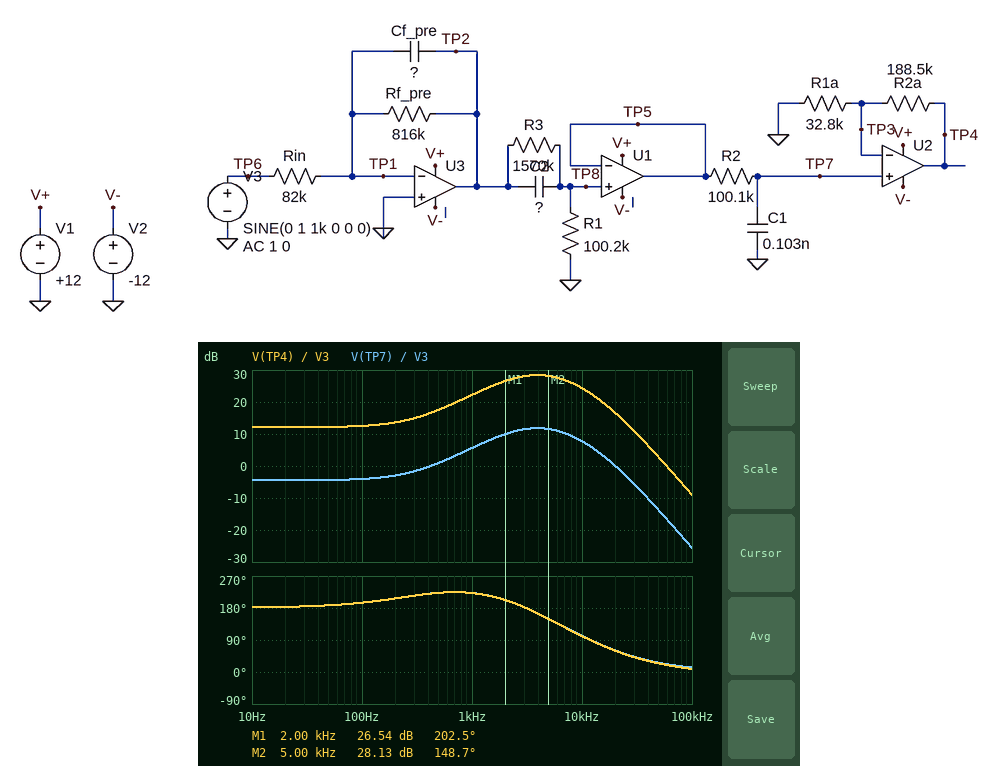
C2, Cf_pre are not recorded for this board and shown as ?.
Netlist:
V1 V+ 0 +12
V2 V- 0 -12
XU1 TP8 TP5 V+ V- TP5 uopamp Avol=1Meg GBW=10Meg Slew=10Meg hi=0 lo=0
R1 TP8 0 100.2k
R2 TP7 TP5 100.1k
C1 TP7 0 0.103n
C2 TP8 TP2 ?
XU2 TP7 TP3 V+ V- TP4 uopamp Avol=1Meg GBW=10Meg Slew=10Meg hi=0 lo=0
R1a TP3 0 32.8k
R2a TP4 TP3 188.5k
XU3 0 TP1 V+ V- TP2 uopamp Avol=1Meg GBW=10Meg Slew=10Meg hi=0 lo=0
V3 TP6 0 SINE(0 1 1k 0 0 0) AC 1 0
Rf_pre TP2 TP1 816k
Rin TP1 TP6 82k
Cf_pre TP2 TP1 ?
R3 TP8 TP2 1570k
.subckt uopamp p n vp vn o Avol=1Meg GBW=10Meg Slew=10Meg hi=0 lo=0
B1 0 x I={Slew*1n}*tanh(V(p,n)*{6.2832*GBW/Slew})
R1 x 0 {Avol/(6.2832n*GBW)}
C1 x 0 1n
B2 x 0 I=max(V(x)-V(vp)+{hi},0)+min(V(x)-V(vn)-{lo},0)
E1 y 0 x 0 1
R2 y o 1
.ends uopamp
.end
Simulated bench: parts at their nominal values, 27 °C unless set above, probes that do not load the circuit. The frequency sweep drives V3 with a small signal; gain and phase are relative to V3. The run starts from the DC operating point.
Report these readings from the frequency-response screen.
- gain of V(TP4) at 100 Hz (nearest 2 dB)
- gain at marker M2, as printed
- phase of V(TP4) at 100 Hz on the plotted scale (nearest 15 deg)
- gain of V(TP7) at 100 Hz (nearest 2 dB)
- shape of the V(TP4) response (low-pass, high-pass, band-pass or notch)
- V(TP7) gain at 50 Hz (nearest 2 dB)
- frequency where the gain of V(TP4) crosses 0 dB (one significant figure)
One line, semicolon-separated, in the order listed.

12 dB; 28.13 dB; 195 deg; -4 dB; band-pass; -4 dB; 60 kHz
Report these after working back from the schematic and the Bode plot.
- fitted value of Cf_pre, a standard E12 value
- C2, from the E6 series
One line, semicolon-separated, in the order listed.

56 pF; 330 pF
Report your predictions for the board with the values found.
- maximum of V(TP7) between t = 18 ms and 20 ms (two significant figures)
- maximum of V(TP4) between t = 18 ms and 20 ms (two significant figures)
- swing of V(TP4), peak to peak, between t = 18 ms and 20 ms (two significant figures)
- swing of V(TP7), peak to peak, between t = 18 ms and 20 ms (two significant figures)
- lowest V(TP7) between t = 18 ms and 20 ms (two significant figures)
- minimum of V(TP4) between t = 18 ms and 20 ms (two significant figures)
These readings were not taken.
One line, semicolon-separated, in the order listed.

1.9 V; 12 V; 24 V; 3.8 V; -1.9 V; -12 V
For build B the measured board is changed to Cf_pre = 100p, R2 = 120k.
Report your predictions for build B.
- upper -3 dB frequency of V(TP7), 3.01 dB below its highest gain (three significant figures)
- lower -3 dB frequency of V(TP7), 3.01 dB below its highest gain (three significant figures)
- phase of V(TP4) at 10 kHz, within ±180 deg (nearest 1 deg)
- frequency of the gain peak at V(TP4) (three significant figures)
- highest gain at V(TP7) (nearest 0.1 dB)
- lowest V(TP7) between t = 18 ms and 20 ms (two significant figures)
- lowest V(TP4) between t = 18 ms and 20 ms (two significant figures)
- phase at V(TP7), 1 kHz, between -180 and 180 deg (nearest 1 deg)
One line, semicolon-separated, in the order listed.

6.98 kHz; 1.11 kHz; 88 deg; 2.93 kHz; 8.6 dB; -1.8 V; -12 V; -150 deg
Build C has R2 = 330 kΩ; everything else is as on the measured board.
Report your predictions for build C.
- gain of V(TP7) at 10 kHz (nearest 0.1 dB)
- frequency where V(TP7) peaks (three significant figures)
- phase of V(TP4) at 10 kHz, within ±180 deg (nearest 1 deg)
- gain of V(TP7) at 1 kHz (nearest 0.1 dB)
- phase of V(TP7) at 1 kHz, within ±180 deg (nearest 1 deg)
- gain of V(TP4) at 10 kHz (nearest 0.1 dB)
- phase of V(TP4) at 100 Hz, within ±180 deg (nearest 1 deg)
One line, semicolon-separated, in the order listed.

1.8 dB; 3.04 kHz; 69 deg; 5.5 dB; -146 deg; 18.4 dB; -166 deg
